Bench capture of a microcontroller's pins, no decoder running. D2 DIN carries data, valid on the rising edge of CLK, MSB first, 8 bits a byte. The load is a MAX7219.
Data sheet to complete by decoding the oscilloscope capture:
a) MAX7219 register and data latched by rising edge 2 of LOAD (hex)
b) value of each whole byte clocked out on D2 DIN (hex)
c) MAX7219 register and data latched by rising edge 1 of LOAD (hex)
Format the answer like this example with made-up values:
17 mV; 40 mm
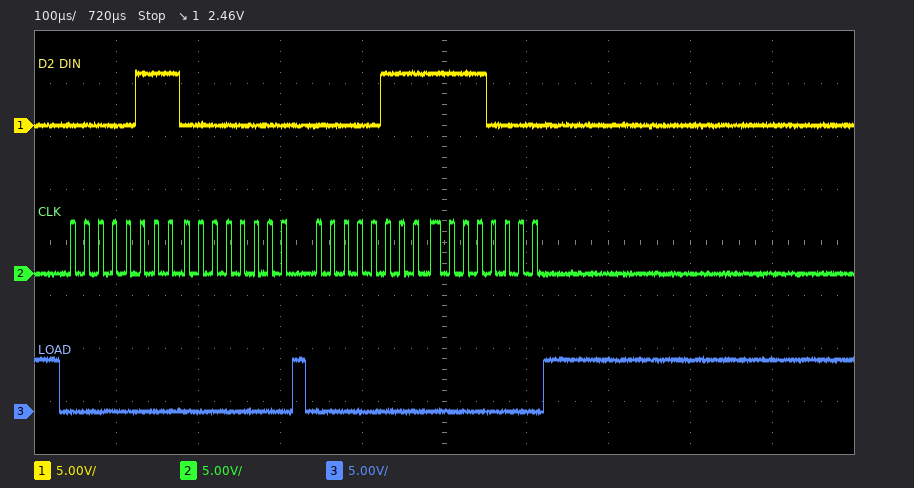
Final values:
register 0x7, data 0xF0; 07 00 07 F0; register 0x7, data 0x00
